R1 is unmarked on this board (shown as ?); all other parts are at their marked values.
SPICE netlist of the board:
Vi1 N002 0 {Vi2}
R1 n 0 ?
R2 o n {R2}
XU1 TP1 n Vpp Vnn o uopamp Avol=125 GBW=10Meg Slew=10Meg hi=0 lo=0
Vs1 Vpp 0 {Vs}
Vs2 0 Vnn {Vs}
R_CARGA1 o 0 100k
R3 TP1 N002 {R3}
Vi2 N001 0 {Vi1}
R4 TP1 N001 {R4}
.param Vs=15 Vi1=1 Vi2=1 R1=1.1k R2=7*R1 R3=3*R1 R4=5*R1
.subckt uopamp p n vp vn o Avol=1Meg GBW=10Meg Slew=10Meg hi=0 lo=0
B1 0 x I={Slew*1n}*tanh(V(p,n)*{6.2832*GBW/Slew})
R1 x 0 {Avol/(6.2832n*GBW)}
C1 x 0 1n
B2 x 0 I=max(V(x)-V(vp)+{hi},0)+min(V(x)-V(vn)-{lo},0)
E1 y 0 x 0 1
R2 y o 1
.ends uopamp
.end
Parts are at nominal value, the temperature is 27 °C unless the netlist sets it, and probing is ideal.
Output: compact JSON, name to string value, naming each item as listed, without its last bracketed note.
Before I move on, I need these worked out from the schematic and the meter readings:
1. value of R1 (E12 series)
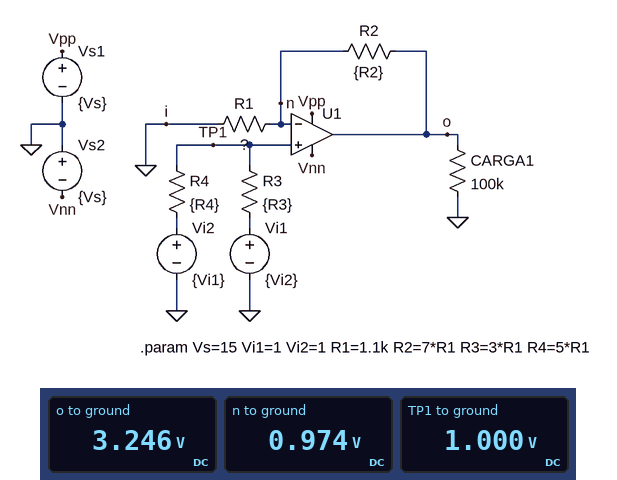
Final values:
{"value of R1": "3.3 kΩ"}
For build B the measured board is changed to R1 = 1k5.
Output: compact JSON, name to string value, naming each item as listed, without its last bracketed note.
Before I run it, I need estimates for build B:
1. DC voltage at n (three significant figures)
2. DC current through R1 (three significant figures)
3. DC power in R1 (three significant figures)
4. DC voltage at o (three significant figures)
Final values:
{"DC voltage at n": "952 mV", "DC current through R1": "635 µA", "DC power in R1": "604 µW", "DC voltage at o": "5.84 V"}
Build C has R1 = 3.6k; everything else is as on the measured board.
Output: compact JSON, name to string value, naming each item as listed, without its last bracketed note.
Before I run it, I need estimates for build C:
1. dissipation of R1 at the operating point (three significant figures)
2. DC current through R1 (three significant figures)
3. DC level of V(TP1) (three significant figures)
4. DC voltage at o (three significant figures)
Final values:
{"dissipation of R1 at the operating point": "264 µW", "DC current through R1": "271 µA", "DC level of V(TP1)": "1.00 V", "DC voltage at o": "3.06 V"}
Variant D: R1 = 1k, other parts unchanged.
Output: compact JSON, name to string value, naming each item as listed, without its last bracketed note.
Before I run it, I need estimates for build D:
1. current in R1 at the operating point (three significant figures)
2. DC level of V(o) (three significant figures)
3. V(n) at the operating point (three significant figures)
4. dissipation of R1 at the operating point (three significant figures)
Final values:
{"current in R1 at the operating point": "931 µA", "DC level of V(o)": "8.10 V", "V(n) at the operating point": "931 mV", "dissipation of R1 at the operating point": "867 µW"}
